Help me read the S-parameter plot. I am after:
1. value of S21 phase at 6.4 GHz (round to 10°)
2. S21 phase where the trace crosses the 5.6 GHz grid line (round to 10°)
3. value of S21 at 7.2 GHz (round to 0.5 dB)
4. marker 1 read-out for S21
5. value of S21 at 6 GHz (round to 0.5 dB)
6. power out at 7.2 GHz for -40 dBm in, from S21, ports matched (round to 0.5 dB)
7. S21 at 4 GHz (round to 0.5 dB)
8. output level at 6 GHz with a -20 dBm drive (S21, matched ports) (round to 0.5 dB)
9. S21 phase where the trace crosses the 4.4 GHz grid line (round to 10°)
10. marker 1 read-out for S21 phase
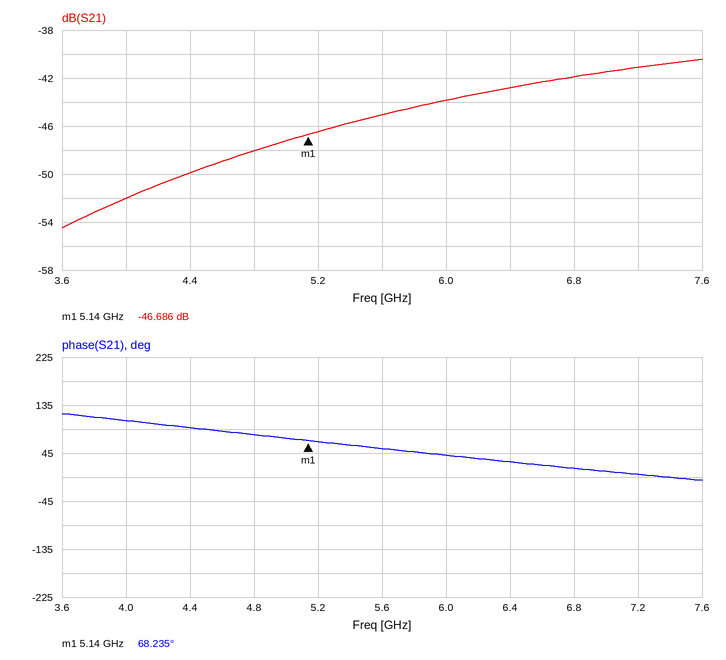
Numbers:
30°
50°
-41.0 dB
-46.686 dB
-44.0 dB
-81.0 dBm
-52.0 dB
-64.0 dBm
90°
68.235°
